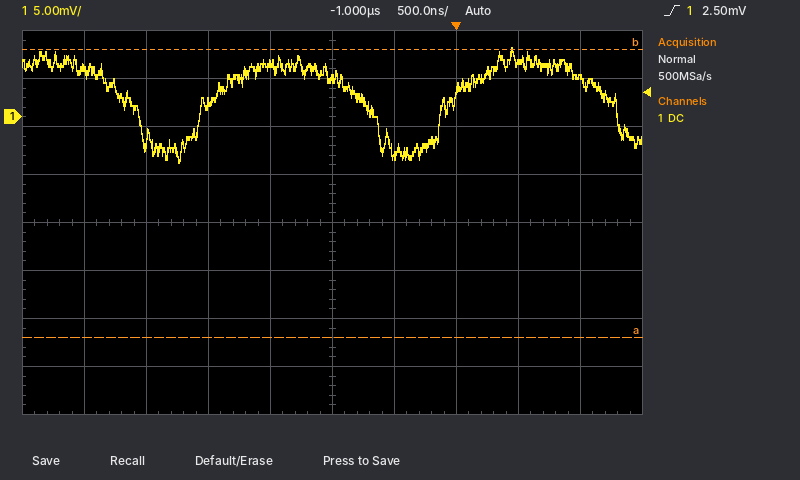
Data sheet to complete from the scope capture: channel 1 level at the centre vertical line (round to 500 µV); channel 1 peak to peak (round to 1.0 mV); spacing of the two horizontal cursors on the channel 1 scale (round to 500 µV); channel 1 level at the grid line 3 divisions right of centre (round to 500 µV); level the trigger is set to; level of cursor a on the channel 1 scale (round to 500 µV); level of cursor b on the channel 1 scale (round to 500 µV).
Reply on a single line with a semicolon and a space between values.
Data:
4.0 mV; 12.0 mV; 30.0 mV; 5.5 mV; 2.50 mV; -23.0 mV; 7.0 mV
